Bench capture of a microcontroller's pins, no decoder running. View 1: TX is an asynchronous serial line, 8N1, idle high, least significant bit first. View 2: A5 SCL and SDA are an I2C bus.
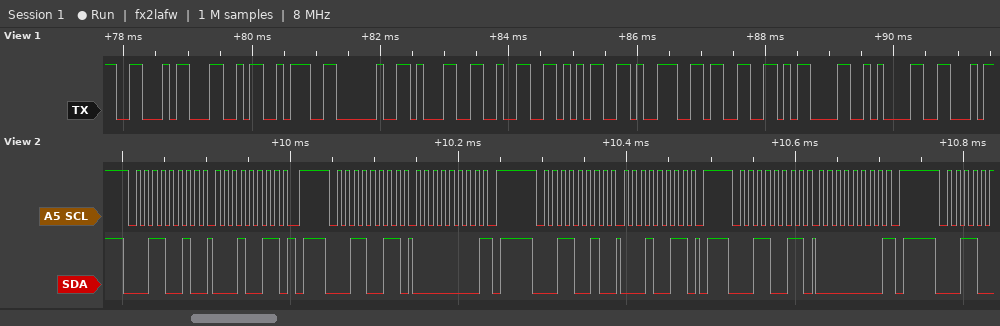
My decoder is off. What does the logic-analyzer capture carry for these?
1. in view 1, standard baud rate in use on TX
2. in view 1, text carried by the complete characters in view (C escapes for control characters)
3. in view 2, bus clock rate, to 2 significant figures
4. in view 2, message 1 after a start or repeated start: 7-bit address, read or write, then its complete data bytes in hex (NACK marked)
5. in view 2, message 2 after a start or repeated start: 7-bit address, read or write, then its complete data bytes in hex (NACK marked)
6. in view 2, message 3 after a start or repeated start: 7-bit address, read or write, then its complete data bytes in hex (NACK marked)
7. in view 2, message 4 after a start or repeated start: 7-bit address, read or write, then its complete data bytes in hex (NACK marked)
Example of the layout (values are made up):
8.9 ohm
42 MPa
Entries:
9600 baud
"FL: 12593\r\nF"
100 kHz
0x19 write: 13
0x19 read: 00 NACK
0x19 write: 13
0x19 read: 00 NACK
